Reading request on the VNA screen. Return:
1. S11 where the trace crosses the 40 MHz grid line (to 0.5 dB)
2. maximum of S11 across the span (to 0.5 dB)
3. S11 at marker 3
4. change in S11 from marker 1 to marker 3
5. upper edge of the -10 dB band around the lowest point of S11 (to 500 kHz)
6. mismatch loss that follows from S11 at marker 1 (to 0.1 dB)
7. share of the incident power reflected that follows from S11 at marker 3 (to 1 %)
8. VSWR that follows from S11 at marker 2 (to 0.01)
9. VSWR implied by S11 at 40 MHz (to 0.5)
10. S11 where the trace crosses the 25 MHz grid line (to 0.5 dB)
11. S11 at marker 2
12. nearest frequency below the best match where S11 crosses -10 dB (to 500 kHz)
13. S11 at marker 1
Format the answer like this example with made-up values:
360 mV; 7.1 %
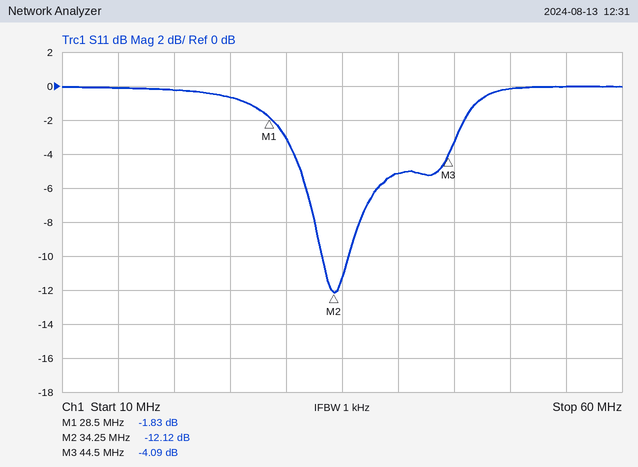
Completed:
-5.0 dB; 0.0 dB; -4.09 dB; -2.26 dB; 35.5 MHz; 4.6 dB; 39 %; 1.66; 3.5; -0.5 dB; -12.12 dB; 33.0 MHz; -1.83 dB
